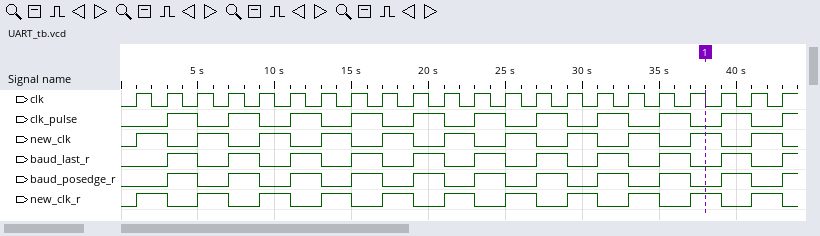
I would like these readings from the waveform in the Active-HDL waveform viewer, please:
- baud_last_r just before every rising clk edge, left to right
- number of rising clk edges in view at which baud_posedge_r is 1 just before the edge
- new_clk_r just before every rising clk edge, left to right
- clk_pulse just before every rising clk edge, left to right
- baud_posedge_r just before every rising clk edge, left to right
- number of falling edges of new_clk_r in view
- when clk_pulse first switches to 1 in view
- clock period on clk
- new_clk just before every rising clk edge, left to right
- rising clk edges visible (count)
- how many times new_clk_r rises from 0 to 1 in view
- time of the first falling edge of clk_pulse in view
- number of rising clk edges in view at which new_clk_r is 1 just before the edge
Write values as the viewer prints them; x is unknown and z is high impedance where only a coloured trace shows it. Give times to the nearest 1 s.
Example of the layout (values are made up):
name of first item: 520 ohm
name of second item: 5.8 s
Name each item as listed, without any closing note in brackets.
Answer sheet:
baud_last_r just before every rising clk edge, left to right: 0 0 1 0 1 0 1 0 1 0 1 0 1 0 1 0 1 0 1 0 1 0
number of rising clk edges in view at which baud_posedge_r is 1 just before the edge: 10
new_clk_r just before every rising clk edge, left to right: 0 1 0 1 0 1 0 1 0 1 0 1 0 1 0 1 0 1 0 1 0 1
clk_pulse just before every rising clk edge, left to right: 0 0 1 0 1 0 1 0 1 0 1 0 1 0 1 0 1 0 1 0 1 0
baud_posedge_r just before every rising clk edge, left to right: 0 0 1 0 1 0 1 0 1 0 1 0 1 0 1 0 1 0 1 0 1 0
number of falling edges of new_clk_r in view: 11
when clk_pulse first switches to 1 in view: 3 s
clock period on clk: 2 s
new_clk just before every rising clk edge, left to right: 0 1 0 1 0 1 0 1 0 1 0 1 0 1 0 1 0 1 0 1 0 1
rising clk edges visible: 22
how many times new_clk_r rises from 0 to 1 in view: 11
time of the first falling edge of clk_pulse in view: 5 s
number of rising clk edges in view at which new_clk_r is 1 just before the edge: 11
